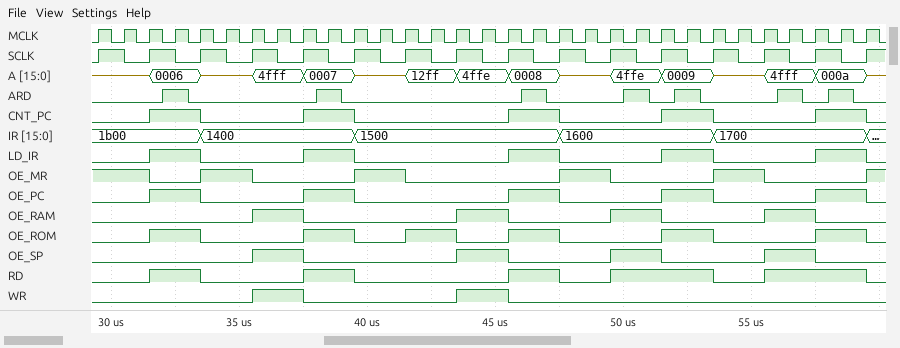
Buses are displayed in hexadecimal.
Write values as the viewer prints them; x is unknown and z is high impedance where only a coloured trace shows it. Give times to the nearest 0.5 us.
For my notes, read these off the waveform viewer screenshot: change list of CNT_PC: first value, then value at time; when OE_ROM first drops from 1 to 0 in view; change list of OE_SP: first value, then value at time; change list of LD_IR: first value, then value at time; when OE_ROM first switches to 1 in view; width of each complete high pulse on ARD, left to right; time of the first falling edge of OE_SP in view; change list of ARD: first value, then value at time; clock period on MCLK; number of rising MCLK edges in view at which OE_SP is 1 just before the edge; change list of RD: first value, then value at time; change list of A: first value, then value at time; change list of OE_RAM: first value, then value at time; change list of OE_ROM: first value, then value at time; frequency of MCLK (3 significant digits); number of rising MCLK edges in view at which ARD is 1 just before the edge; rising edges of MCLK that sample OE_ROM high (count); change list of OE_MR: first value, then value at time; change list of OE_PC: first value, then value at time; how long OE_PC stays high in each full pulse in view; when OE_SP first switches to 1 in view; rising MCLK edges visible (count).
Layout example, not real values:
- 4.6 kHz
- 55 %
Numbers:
- 0, 1 at 31.5 us, 0 at 33.5 us, 1 at 37.5 us, 0 at 39.5 us, 1 at 45.5 us, 0 at 47.5 us, 1 at 51.5 us, 0 at 53.5 us, 1 at 57.5 us, 0 at 59.5 us
- 33.5 us
- 0, 1 at 35.5 us, 0 at 37.5 us, 1 at 43.5 us, 0 at 45.5 us, 1 at 49.5 us, 0 at 51.5 us, 1 at 55.5 us, 0 at 57.5 us
- 0, 1 at 31.5 us, 0 at 33.5 us, 1 at 37.5 us, 0 at 39.5 us, 1 at 45.5 us, 0 at 47.5 us, 1 at 51.5 us, 0 at 53.5 us, 1 at 57.5 us, 0 at 59.5 us
- 31.5 us
- 1 us, 1 us, 1 us, 1 us, 1 us, 1 us, 1 us
- 37.5 us
- 0, 1 at 32 us, 0 at 33 us, 1 at 38 us, 0 at 39 us, 1 at 46 us, 0 at 47 us, 1 at 50 us, 0 at 51 us, 1 at 52 us, 0 at 53 us, 1 at 56 us, 0 at 57 us, 1 at 58 us, 0 at 59 us
- 1 us
- 8
- 0, 1 at 31.5 us, 0 at 33.5 us, 1 at 37.5 us, 0 at 39.5 us, 1 at 45.5 us, 0 at 47.5 us, 1 at 49.5 us, 0 at 53.5 us, 1 at 55.5 us, 0 at 59.5 us
- z, 0006 at 31.5 us, z at 33.5 us, 4fff at 35.5 us, 0007 at 37.5 us, z at 39.5 us, 12ff at 41.5 us, 4ffe at 43.5 us, 0008 at 45.5 us, z at 47.5 us, 4ffe at 49.5 us, 0009 at 51.5 us, z at 53.5 us, 4fff at 55.5 us, 000a at 57.5 us, z at 59.5 us
- 0, 1 at 35.5 us, 0 at 37.5 us, 1 at 43.5 us, 0 at 45.5 us, 1 at 49.5 us, 0 at 51.5 us, 1 at 55.5 us, 0 at 57.5 us
- 0, 1 at 31.5 us, 0 at 33.5 us, 1 at 37.5 us, 0 at 39.5 us, 1 at 41.5 us, 0 at 43.5 us, 1 at 45.5 us, 0 at 47.5 us, 1 at 51.5 us, 0 at 53.5 us, 1 at 57.5 us, 0 at 59.5 us
- 1.00 MHz
- 7
- 12
- 1, 0 at 31.5 us, 1 at 33.5 us, 0 at 35.5 us, 1 at 39.5 us, 0 at 41.5 us, 1 at 47.5 us, 0 at 49.5 us, 1 at 53.5 us, 0 at 55.5 us, 1 at 59.5 us
- 0, 1 at 31.5 us, 0 at 33.5 us, 1 at 37.5 us, 0 at 39.5 us, 1 at 45.5 us, 0 at 47.5 us, 1 at 51.5 us, 0 at 53.5 us, 1 at 57.5 us, 0 at 59.5 us
- 2 us, 2 us, 2 us, 2 us, 2 us
- 35.5 us
- 31
